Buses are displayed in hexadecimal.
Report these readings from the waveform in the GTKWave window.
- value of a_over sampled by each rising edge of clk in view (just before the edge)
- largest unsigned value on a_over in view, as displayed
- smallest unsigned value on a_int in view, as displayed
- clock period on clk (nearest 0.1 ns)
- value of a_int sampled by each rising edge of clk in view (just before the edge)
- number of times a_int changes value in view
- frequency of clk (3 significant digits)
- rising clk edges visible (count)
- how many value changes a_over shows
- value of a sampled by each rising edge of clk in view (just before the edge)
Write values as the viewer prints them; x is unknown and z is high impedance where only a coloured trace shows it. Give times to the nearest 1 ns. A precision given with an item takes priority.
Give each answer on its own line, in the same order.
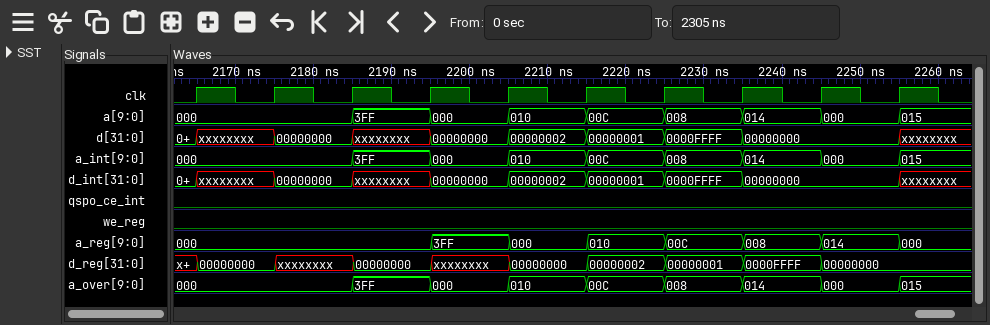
000, 000, 000, 3FF, 000, 010, 00C, 008, 014, 000
3FF
000
10 ns
000, 000, 000, 3FF, 000, 010, 00C, 008, 014, 000
8
100 MHz
10
8
000, 000, 000, 3FF, 000, 010, 00C, 008, 014, 000
